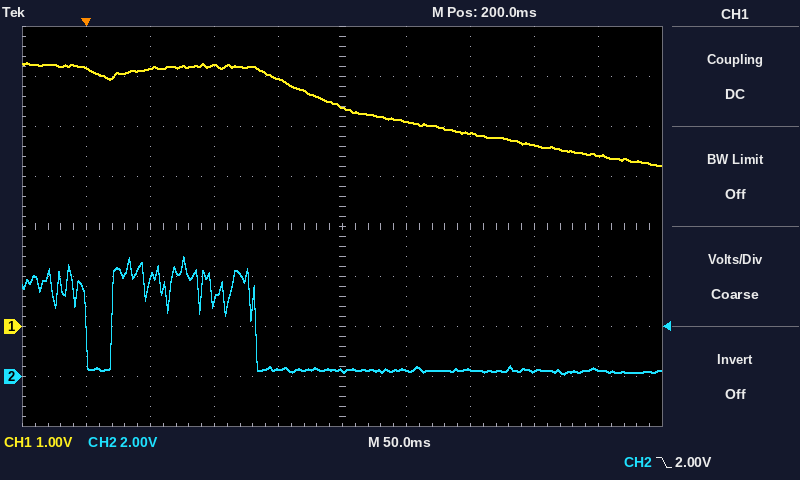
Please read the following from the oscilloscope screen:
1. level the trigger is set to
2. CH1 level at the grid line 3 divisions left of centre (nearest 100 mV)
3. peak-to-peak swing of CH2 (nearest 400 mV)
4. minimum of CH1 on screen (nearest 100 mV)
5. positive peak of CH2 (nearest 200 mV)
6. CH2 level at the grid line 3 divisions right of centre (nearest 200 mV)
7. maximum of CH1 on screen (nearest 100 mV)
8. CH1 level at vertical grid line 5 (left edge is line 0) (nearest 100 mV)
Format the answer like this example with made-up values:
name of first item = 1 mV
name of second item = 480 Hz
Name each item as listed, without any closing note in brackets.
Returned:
level the trigger is set to = 2.00 V
CH1 level at the grid line 3 divisions left of centre = 5.2 V
peak-to-peak swing of CH2 = 4.8 V
minimum of CH1 on screen = 3.2 V
positive peak of CH2 = 4.8 V
CH2 level at the grid line 3 divisions right of centre = 200 mV
maximum of CH1 on screen = 5.3 V
CH1 level at vertical grid line 5 (left edge is line 0) = 4.4 V
